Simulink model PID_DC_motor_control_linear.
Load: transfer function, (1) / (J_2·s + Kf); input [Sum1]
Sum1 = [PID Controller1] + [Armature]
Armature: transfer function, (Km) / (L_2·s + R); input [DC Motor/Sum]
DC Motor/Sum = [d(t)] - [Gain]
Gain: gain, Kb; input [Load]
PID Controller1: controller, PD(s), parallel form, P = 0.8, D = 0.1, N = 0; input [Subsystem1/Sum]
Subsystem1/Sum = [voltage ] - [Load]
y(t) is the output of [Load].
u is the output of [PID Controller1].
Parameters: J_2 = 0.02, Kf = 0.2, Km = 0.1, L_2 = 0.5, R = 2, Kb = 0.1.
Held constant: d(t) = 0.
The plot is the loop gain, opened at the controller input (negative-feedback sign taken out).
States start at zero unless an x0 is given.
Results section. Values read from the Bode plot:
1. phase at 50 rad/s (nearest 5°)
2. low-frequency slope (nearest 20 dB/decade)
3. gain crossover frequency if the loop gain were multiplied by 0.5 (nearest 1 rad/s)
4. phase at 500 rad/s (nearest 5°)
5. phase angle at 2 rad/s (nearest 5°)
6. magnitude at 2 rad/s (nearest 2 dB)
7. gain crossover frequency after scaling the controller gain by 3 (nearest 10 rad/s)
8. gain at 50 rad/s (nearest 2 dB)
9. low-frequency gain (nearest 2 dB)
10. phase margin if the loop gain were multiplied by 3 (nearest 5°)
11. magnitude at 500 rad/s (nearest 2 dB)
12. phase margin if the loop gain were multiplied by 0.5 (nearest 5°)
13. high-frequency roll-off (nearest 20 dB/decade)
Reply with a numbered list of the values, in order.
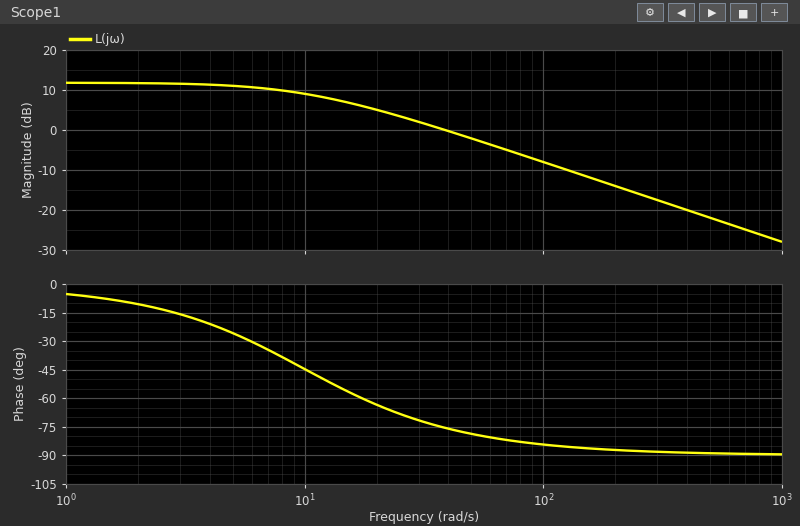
1. -80°
2. 0 dB/decade
3. 17 rad/s
4. -90°
5. -10°
6. 12 dB
7. 120 rad/s
8. -2 dB
9. 12 dB
10. 95°
11. -22 dB
12. 120°
13. -20 dB/decade
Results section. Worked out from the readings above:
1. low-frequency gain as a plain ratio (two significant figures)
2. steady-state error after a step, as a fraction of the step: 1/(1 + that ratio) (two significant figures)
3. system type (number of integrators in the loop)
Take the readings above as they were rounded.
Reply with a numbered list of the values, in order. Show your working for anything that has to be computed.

1. 10^(12 / 20) = 4.0
2. 1 / (1 + 4) = 0.20
3. 0
